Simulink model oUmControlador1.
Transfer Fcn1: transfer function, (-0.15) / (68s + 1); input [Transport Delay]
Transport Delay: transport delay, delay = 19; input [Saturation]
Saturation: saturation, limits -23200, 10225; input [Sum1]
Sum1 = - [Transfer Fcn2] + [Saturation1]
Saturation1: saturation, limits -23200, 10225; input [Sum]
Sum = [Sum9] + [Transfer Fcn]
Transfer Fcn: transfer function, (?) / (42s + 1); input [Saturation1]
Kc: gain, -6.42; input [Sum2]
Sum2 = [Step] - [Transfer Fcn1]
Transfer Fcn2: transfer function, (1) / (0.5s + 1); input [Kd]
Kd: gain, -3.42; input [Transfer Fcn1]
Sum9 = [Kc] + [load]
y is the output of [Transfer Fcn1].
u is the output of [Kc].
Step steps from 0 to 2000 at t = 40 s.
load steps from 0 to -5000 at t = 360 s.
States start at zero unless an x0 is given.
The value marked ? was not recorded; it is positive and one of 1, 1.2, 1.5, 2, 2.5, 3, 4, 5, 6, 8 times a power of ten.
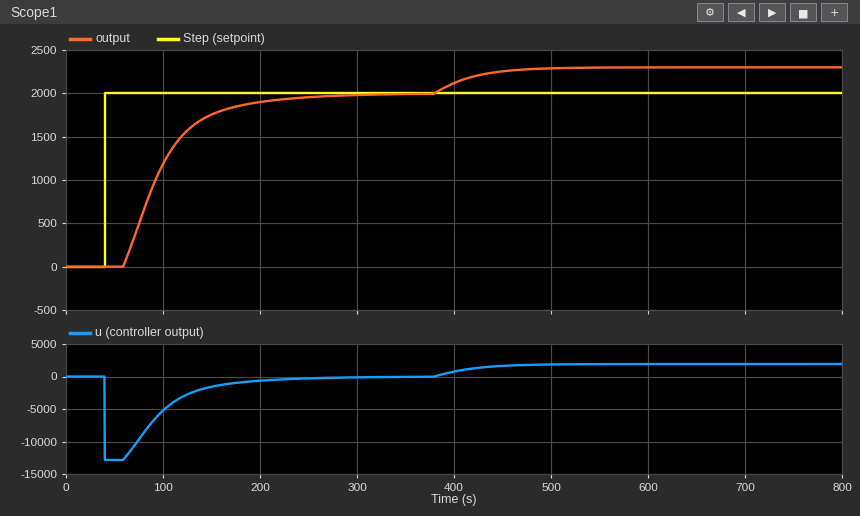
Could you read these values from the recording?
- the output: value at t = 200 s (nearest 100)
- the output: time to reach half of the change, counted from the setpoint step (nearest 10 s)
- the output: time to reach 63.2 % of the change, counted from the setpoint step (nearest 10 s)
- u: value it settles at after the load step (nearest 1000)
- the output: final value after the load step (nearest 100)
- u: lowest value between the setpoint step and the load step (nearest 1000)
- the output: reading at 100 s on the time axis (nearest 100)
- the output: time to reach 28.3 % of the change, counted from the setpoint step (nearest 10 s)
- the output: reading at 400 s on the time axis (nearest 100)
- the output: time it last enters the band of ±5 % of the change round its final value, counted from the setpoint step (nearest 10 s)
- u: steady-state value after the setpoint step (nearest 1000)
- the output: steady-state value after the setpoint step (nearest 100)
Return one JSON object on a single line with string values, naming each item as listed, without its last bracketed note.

{"the output: value at t = 200 s": "1900", "the output: time to reach half of the change, counted from the setpoint step": "50 s", "the output: time to reach 63.2 % of the change, counted from the setpoint step": "60 s", "u: value it settles at after the load step": "2000", "the output: final value after the load step": "2300", "u: lowest value between the setpoint step and the load step": "-13000", "the output: reading at 100 s on the time axis": "1200", "the output: time to reach 28.3 % of the change, counted from the setpoint step": "40 s", "the output: reading at 400 s on the time axis": "2100", "the output: time it last enters the band of ±5 % of the change round its final value, counted from the setpoint step": "160 s", "u: steady-state value after the setpoint step": "0", "the output: steady-state value after the setpoint step": "2000"}
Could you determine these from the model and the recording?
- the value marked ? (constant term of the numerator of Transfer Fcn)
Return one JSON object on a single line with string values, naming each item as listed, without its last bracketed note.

{"the value marked ?": "1"}
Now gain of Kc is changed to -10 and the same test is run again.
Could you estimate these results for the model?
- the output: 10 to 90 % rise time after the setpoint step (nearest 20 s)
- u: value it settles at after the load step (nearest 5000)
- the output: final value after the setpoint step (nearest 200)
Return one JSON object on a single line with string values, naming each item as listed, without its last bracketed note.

{"the output: 10 to 90 % rise time after the setpoint step": "60 s", "u: value it settles at after the load step": "5000", "the output: final value after the setpoint step": "2000"}
